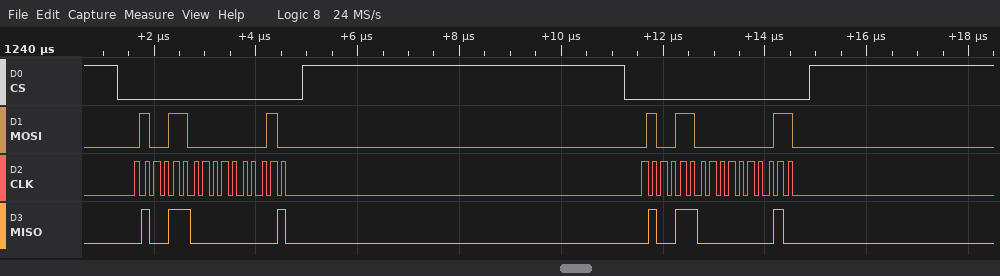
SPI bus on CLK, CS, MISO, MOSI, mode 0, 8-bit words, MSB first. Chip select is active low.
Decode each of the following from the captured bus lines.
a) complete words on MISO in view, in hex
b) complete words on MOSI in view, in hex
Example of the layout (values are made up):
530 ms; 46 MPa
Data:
4C, 01, 4C, 02; 4C, 02, 4C, 03
